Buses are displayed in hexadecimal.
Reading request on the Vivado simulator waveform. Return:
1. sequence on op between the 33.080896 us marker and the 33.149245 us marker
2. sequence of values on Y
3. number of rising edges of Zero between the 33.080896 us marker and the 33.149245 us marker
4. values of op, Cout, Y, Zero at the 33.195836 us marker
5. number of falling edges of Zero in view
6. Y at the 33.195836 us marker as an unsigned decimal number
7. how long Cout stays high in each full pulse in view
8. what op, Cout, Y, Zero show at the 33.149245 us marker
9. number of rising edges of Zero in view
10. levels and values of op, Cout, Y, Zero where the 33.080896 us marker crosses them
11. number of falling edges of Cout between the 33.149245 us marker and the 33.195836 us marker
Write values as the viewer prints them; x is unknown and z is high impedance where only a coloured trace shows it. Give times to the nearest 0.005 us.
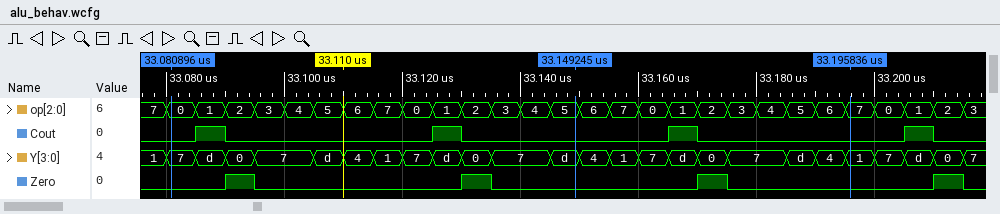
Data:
0, 1, 2, 3, 4, 5, 6, 7, 0, 1, 2, 3, 4, 5
1, 7, d, 0, 7, d, 4, 1, 7, d, 0, 7, d, 4, 1, 7, d, 0, 7, d, 4, 1, 7, d, 0, 7
2
op=7, Cout=0, Y=1, Zero=0
4
1
0.005 us, 0.005 us, 0.005 us, 0.005 us
op=5, Cout=0, Y=d, Zero=0
4
op=0, Cout=0, Y=7, Zero=0
1
